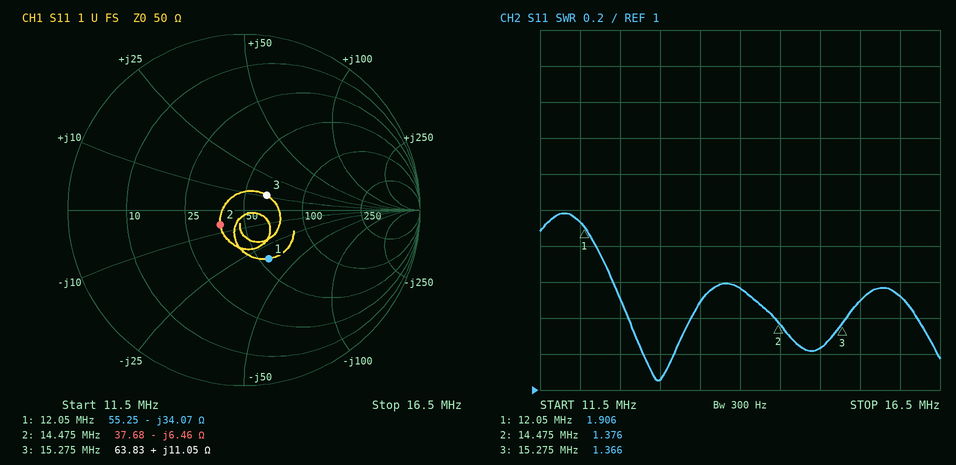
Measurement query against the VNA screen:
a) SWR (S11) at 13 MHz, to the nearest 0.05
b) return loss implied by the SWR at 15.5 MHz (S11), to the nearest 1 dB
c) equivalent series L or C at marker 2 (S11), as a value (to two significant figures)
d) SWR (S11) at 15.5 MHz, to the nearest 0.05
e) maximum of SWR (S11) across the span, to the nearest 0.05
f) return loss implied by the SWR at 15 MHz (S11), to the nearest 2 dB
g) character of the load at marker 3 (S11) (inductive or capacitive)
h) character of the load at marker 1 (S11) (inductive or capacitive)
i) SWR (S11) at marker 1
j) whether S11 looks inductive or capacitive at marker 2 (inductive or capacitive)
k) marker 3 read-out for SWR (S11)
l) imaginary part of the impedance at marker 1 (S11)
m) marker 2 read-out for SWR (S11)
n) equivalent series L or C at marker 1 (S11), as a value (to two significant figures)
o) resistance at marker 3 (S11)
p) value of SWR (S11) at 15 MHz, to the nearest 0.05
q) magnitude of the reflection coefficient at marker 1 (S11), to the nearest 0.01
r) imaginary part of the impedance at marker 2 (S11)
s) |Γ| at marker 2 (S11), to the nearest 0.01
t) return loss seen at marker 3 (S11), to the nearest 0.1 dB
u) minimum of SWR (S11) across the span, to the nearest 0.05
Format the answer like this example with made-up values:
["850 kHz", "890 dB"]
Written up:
["1.05", "14 dB", "1.7 nF", "1.50", "2.00", "20 dB", "inductive", "capacitive", "1.906", "capacitive", "1.366", "-34.07 Ω", "1.376", "390 pF", "63.83 Ω", "1.25", "0.31", "-6.46 Ω", "0.16", "16.2 dB", "1.05"]
